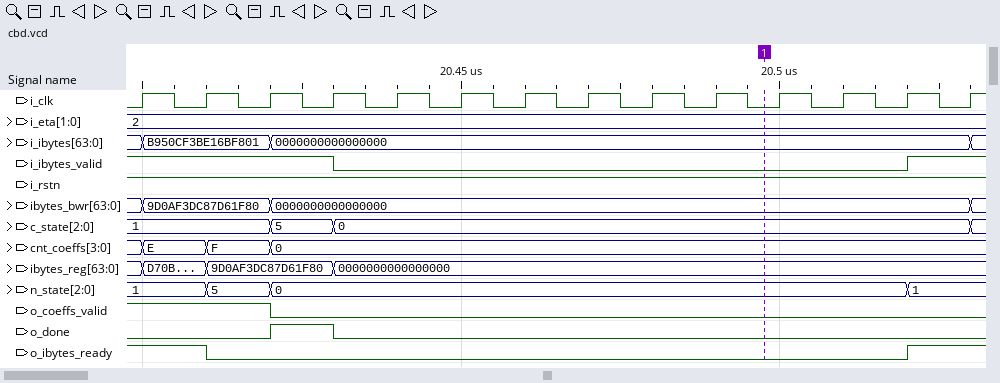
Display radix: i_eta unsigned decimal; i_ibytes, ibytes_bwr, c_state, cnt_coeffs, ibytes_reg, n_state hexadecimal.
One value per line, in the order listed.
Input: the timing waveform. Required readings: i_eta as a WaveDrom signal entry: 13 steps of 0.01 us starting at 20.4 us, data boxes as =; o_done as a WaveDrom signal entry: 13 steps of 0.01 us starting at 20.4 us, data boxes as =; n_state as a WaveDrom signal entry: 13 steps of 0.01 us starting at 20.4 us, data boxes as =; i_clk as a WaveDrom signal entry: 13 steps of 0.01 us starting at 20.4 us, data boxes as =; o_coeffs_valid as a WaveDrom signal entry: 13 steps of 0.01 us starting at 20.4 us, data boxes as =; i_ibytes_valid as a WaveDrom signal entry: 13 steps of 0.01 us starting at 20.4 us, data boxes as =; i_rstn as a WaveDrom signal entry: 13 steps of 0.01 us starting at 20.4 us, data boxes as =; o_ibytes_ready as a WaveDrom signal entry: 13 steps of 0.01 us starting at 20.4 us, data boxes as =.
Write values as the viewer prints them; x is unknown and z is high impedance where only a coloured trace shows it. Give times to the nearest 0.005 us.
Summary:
{name: 'i_eta', wave: '=............', data: '2'}
{name: 'o_done', wave: '0.10.........'}
{name: 'n_state', wave: '===.........=', data: '1 5 0 1'}
{name: 'i_clk', wave: 'p............'}
{name: 'o_coeffs_valid', wave: '1.0..........'}
{name: 'i_ibytes_valid', wave: '1..0........1'}
{name: 'i_rstn', wave: '1............'}
{name: 'o_ibytes_ready', wave: '10..........1'}
